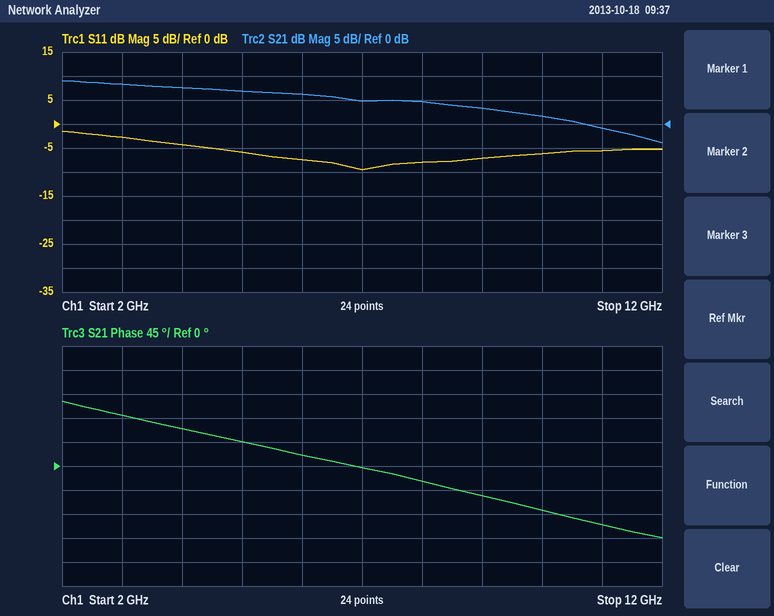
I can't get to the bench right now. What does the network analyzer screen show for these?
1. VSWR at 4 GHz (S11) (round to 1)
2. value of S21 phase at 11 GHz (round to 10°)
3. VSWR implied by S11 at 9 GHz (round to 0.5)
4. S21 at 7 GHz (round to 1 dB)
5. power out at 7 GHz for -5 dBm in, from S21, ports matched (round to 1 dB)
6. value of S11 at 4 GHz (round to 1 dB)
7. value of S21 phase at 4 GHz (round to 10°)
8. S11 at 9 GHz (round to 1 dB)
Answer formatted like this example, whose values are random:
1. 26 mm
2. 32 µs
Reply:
1. 4
2. -110°
3. 2.5
4. 5 dB
5. 0 dBm
6. -4 dB
7. 70°
8. -7 dB
